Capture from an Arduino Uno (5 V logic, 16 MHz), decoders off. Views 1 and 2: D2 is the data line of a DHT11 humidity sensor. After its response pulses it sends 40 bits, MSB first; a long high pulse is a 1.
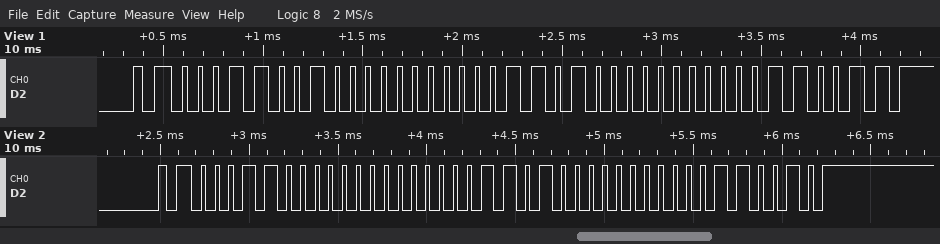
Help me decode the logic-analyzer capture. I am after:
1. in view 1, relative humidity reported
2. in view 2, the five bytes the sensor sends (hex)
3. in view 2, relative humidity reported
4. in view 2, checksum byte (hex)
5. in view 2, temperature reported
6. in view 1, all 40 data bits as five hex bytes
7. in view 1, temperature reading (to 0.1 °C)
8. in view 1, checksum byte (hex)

25 %
18 00 1A 00 32
24 %
0x32
26.0 °C
19 00 1A 00 33
26.0 °C
0x33
